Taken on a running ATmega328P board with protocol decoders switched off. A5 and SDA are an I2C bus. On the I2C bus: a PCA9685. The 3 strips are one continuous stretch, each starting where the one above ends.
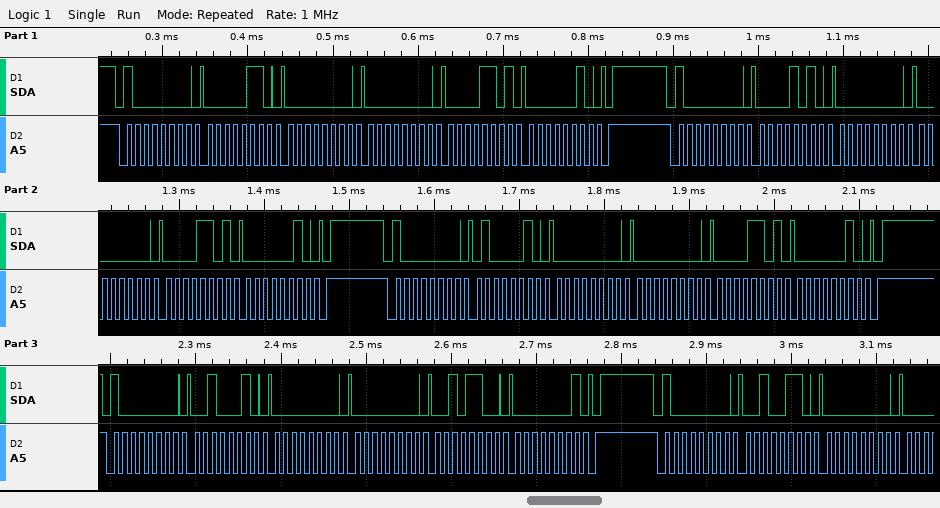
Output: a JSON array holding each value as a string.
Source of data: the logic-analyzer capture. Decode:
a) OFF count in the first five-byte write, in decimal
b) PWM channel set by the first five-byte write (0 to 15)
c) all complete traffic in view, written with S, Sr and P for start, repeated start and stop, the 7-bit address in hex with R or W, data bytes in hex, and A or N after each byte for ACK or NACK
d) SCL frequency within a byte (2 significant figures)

["525", "0", "S 40W A 06 A 00 A 00 A 0D A 02 A P S 40W A 0A A 00 A 00 A 0D A 02 A P S 40W A 42 A 00 A 00 A 0D A 02 A P S 40W A 22 A 00 A 00 A 2C A 01 A P S 40W A 26 A 00 A", "100 kHz"]
